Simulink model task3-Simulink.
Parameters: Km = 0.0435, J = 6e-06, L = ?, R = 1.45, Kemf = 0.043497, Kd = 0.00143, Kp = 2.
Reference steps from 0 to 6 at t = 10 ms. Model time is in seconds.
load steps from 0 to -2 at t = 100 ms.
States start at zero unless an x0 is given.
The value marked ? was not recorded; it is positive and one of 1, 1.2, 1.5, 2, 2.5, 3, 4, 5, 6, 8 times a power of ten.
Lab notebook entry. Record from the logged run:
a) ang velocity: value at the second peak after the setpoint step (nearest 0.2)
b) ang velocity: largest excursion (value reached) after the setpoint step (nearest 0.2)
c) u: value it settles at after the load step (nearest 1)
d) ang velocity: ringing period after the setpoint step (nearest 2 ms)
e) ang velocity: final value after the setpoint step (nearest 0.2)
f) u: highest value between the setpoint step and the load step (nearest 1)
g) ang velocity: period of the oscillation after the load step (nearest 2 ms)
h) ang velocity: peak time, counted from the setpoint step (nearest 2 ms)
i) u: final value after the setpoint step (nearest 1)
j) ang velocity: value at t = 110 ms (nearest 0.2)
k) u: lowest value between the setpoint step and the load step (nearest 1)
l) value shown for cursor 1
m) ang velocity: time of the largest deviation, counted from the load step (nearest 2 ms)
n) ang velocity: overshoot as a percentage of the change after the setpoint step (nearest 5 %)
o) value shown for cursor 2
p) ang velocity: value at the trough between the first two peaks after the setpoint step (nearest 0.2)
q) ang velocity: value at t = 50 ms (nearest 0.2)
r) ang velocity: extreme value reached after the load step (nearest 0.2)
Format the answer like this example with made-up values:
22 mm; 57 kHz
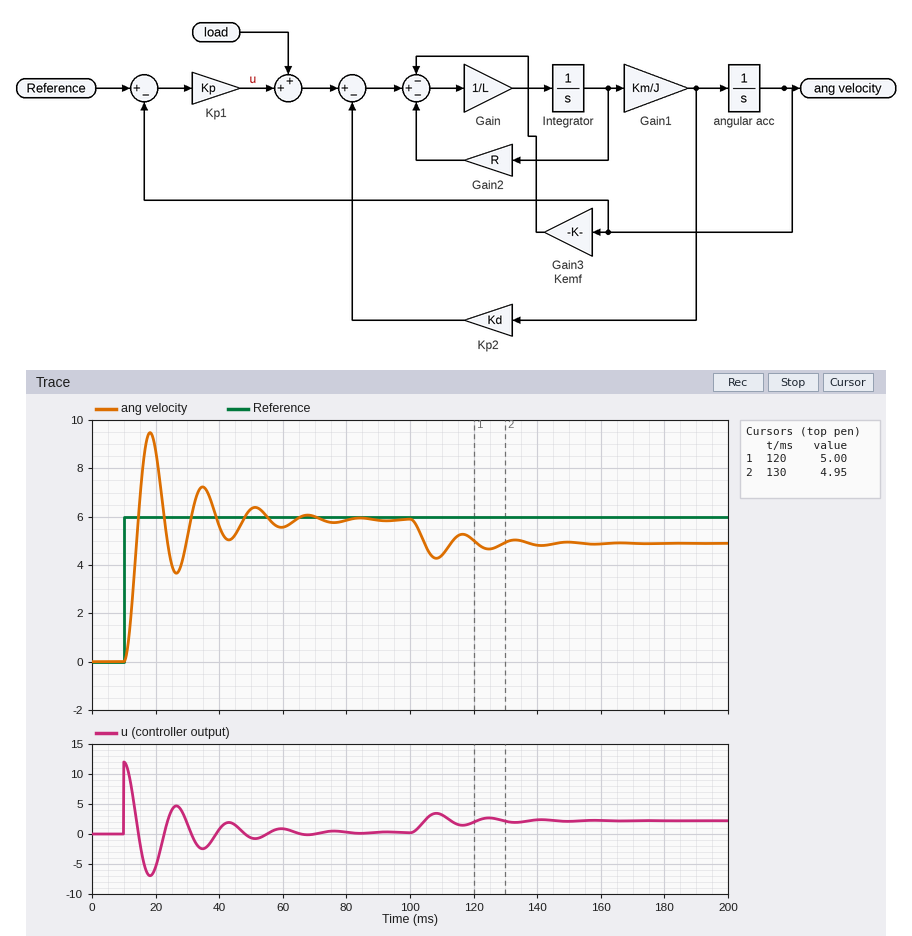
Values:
7.2; 9.4; 2; 16 ms; 5.8; 12; 16 ms; 8 ms; 0; 4.4; -7; 5.00; 8 ms; 60 %; 4.95; 3.6; 6.4; 4.2
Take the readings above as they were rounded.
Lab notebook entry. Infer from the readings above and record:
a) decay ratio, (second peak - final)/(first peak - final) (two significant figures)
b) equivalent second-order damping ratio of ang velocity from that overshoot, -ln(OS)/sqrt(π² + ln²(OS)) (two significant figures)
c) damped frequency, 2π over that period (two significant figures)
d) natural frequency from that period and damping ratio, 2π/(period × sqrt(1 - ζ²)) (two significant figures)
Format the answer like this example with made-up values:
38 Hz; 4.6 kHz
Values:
0.39; 0.16; 0.39 rad/ms; 0.40 rad/ms
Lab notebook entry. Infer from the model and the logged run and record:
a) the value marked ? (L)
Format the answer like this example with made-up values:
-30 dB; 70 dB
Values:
0.1
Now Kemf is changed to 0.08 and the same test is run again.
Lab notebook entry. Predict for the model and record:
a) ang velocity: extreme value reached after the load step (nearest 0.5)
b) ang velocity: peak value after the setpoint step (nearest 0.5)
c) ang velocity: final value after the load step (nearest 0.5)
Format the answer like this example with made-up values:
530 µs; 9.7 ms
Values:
4.0; 9.5; 5.0
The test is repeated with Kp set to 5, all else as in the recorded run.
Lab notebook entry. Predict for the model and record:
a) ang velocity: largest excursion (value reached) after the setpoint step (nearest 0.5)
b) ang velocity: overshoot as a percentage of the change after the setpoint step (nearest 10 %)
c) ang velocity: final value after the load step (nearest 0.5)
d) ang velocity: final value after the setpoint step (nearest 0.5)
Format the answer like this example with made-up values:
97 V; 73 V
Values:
10.5; 70 %; 5.5; 6.0
